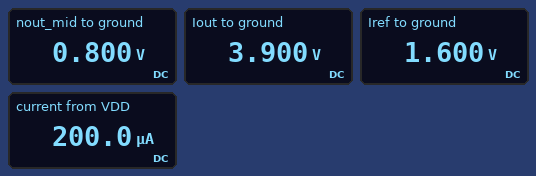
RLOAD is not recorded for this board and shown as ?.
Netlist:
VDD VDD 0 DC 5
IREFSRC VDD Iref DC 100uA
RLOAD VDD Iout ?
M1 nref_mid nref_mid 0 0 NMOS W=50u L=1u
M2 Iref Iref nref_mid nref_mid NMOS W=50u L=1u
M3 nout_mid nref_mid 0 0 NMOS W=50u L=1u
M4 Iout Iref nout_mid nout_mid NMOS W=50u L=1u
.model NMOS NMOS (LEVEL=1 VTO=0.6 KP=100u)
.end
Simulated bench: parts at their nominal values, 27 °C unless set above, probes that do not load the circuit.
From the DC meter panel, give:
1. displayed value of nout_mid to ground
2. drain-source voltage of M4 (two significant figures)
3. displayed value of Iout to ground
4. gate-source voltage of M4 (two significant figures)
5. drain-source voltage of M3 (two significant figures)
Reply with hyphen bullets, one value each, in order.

- 0.800 V
- 3.1 V
- 3.900 V
- 800 mV
- 800 mV
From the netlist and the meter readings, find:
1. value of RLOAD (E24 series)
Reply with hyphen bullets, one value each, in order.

- 11 kΩ
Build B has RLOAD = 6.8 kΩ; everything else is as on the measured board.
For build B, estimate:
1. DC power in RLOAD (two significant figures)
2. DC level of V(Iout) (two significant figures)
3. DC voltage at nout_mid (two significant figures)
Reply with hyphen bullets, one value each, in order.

- 68 µW
- 4.3 V
- 800 mV
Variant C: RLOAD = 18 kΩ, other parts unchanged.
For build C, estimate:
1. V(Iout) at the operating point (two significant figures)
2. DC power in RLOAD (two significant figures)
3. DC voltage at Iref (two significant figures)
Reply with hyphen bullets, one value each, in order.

- 3.2 V
- 180 µW
- 1.6 V
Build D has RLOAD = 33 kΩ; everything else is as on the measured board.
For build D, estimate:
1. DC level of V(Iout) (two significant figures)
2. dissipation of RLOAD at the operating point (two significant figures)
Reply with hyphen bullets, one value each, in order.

- 1.7 V
- 330 µW
